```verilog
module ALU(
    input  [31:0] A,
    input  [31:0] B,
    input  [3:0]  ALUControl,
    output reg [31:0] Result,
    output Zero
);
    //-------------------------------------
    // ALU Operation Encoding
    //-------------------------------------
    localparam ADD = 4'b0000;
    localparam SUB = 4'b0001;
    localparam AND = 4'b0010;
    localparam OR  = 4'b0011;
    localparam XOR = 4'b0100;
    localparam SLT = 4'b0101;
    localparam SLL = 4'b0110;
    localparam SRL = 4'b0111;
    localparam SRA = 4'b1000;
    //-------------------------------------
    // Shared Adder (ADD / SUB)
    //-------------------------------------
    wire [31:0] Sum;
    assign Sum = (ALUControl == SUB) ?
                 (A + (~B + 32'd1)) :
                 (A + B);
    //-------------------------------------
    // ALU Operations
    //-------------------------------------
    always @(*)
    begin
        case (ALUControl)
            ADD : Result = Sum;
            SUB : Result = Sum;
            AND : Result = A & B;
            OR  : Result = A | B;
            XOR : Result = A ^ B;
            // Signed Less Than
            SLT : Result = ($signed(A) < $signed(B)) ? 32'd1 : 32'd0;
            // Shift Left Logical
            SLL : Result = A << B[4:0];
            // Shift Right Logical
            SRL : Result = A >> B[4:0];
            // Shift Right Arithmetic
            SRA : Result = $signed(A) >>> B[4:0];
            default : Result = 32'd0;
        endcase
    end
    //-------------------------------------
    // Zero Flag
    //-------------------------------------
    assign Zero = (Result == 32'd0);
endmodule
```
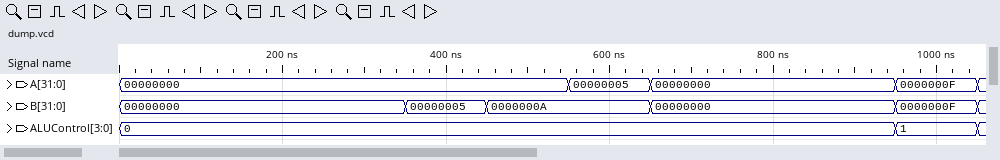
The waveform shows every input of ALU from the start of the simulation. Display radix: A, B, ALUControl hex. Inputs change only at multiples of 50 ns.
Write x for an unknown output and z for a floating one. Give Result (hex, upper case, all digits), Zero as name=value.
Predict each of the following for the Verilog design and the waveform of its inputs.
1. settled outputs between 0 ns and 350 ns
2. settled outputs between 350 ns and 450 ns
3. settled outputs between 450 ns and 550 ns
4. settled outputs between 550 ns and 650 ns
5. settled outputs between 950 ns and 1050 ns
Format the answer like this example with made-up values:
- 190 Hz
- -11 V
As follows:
- Result=00000000, Zero=1
- Result=00000005, Zero=0
- Result=0000000A, Zero=0
- Result=0000000F, Zero=0
- Result=00000000, Zero=1
